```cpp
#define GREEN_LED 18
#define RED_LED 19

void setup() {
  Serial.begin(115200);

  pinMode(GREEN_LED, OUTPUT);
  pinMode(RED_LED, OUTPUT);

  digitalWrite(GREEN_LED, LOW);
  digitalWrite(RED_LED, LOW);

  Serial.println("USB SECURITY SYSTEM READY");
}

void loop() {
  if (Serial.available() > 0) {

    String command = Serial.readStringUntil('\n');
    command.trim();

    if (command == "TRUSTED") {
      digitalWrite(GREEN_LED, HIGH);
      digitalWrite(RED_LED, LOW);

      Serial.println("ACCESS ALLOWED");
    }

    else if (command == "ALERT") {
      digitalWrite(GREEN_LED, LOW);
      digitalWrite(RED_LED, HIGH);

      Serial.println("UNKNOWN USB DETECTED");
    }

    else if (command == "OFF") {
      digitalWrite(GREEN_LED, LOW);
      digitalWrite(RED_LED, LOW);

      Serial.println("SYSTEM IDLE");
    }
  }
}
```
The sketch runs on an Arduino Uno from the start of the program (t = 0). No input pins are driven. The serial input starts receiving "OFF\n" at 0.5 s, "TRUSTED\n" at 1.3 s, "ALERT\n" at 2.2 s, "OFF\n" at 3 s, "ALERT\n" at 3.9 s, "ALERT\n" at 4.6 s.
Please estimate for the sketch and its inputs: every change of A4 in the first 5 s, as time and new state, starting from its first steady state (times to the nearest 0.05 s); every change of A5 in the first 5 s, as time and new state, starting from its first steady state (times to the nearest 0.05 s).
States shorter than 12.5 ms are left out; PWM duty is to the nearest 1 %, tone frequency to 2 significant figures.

0 s low; 1.3 s high; 2.2 s low
0 s low; 2.2 s high; 3 s low; 3.9 s high
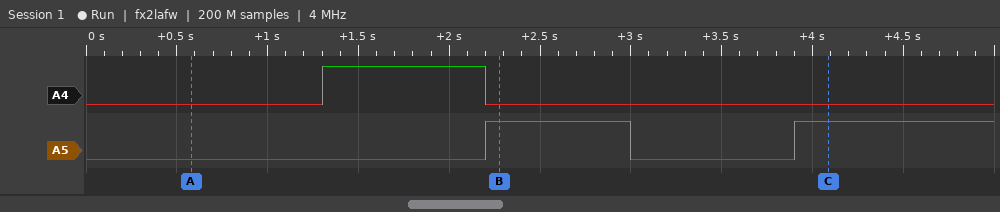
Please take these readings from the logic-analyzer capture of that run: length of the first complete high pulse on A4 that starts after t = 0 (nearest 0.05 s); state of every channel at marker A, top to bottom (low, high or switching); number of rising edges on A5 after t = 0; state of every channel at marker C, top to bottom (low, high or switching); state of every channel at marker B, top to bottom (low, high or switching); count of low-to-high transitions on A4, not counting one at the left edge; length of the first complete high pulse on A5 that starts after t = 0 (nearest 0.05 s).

0.90 s
A4 low, A5 low
2
A4 low, A5 high
A4 low, A5 high
1
0.80 s
